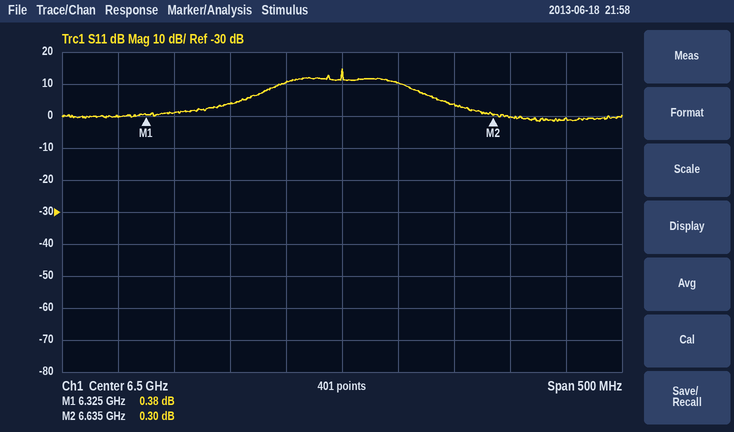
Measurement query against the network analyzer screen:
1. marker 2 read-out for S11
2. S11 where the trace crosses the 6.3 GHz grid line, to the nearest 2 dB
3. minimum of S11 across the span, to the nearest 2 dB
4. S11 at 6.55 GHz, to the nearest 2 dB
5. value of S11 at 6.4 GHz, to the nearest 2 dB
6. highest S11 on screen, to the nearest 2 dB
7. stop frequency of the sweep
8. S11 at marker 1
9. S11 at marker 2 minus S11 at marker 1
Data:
0.30 dB
0 dB
-2 dB
10 dB
4 dB
14 dB
6.75 GHz
0.38 dB
-0.08 dB
